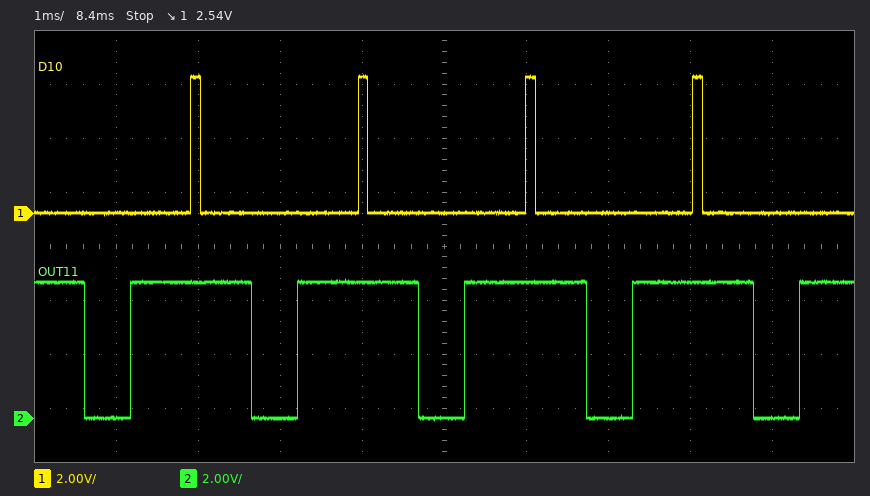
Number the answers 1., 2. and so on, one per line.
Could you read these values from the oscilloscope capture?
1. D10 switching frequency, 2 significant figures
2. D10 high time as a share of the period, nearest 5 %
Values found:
1. 490 Hz
2. 5 %
